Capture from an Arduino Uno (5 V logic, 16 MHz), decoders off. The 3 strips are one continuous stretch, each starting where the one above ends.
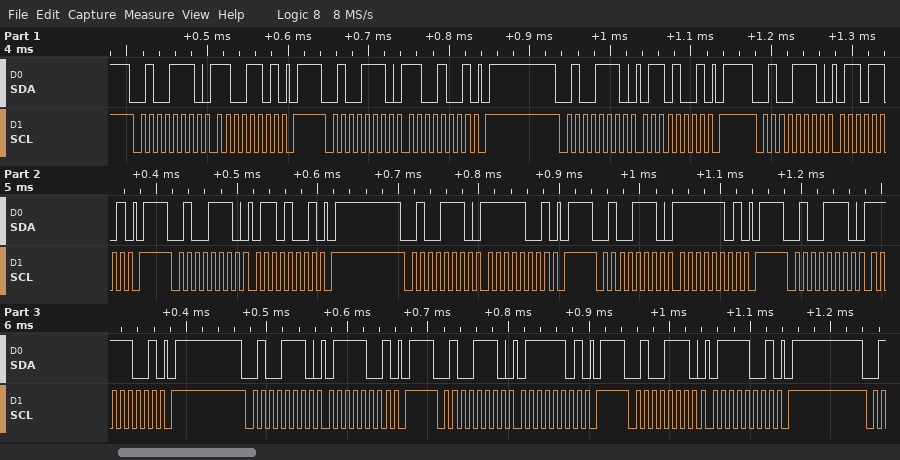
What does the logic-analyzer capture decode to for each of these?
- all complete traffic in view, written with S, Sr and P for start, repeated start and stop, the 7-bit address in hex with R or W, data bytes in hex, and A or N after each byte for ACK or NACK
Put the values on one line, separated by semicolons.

S 27W A CD A P S 27W A C9 A P S 27W A 69 A P S 27W A 6D A P S 27W A 69 A P S 27W A F9 A P S 27W A FD A P S 27W A F9 A P S 27W A 79 A P S 27W A 7D A P S 27W A 79 A P
